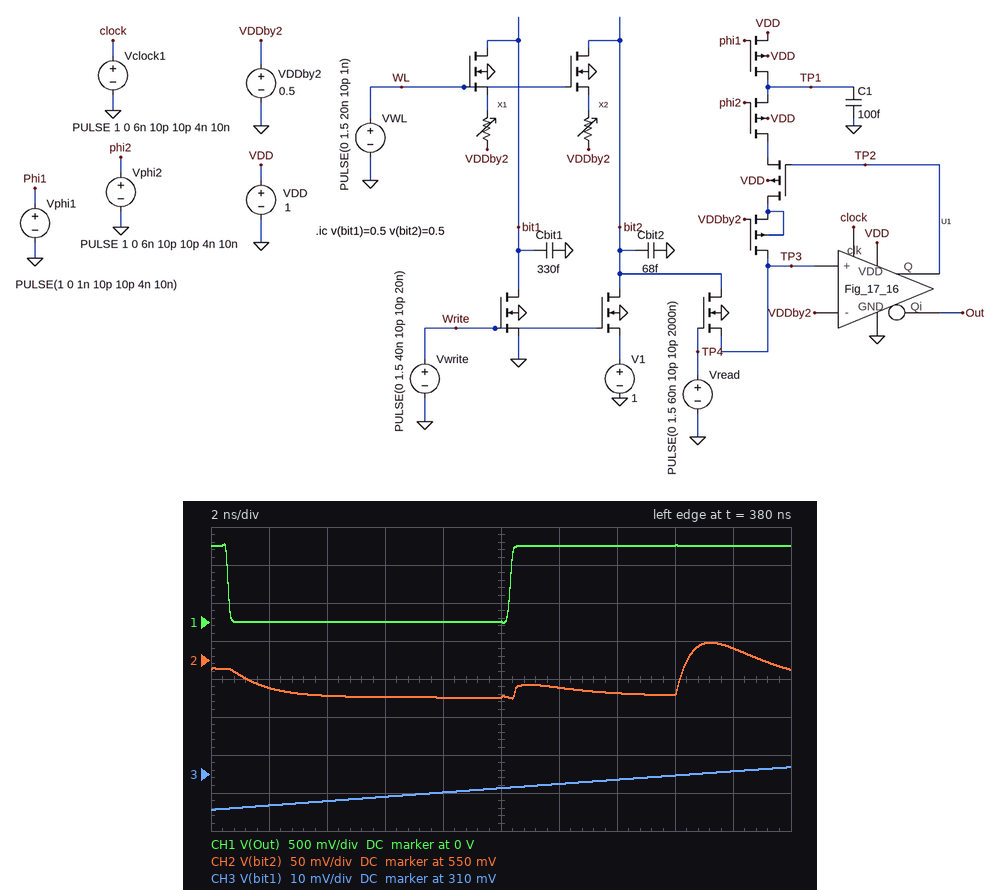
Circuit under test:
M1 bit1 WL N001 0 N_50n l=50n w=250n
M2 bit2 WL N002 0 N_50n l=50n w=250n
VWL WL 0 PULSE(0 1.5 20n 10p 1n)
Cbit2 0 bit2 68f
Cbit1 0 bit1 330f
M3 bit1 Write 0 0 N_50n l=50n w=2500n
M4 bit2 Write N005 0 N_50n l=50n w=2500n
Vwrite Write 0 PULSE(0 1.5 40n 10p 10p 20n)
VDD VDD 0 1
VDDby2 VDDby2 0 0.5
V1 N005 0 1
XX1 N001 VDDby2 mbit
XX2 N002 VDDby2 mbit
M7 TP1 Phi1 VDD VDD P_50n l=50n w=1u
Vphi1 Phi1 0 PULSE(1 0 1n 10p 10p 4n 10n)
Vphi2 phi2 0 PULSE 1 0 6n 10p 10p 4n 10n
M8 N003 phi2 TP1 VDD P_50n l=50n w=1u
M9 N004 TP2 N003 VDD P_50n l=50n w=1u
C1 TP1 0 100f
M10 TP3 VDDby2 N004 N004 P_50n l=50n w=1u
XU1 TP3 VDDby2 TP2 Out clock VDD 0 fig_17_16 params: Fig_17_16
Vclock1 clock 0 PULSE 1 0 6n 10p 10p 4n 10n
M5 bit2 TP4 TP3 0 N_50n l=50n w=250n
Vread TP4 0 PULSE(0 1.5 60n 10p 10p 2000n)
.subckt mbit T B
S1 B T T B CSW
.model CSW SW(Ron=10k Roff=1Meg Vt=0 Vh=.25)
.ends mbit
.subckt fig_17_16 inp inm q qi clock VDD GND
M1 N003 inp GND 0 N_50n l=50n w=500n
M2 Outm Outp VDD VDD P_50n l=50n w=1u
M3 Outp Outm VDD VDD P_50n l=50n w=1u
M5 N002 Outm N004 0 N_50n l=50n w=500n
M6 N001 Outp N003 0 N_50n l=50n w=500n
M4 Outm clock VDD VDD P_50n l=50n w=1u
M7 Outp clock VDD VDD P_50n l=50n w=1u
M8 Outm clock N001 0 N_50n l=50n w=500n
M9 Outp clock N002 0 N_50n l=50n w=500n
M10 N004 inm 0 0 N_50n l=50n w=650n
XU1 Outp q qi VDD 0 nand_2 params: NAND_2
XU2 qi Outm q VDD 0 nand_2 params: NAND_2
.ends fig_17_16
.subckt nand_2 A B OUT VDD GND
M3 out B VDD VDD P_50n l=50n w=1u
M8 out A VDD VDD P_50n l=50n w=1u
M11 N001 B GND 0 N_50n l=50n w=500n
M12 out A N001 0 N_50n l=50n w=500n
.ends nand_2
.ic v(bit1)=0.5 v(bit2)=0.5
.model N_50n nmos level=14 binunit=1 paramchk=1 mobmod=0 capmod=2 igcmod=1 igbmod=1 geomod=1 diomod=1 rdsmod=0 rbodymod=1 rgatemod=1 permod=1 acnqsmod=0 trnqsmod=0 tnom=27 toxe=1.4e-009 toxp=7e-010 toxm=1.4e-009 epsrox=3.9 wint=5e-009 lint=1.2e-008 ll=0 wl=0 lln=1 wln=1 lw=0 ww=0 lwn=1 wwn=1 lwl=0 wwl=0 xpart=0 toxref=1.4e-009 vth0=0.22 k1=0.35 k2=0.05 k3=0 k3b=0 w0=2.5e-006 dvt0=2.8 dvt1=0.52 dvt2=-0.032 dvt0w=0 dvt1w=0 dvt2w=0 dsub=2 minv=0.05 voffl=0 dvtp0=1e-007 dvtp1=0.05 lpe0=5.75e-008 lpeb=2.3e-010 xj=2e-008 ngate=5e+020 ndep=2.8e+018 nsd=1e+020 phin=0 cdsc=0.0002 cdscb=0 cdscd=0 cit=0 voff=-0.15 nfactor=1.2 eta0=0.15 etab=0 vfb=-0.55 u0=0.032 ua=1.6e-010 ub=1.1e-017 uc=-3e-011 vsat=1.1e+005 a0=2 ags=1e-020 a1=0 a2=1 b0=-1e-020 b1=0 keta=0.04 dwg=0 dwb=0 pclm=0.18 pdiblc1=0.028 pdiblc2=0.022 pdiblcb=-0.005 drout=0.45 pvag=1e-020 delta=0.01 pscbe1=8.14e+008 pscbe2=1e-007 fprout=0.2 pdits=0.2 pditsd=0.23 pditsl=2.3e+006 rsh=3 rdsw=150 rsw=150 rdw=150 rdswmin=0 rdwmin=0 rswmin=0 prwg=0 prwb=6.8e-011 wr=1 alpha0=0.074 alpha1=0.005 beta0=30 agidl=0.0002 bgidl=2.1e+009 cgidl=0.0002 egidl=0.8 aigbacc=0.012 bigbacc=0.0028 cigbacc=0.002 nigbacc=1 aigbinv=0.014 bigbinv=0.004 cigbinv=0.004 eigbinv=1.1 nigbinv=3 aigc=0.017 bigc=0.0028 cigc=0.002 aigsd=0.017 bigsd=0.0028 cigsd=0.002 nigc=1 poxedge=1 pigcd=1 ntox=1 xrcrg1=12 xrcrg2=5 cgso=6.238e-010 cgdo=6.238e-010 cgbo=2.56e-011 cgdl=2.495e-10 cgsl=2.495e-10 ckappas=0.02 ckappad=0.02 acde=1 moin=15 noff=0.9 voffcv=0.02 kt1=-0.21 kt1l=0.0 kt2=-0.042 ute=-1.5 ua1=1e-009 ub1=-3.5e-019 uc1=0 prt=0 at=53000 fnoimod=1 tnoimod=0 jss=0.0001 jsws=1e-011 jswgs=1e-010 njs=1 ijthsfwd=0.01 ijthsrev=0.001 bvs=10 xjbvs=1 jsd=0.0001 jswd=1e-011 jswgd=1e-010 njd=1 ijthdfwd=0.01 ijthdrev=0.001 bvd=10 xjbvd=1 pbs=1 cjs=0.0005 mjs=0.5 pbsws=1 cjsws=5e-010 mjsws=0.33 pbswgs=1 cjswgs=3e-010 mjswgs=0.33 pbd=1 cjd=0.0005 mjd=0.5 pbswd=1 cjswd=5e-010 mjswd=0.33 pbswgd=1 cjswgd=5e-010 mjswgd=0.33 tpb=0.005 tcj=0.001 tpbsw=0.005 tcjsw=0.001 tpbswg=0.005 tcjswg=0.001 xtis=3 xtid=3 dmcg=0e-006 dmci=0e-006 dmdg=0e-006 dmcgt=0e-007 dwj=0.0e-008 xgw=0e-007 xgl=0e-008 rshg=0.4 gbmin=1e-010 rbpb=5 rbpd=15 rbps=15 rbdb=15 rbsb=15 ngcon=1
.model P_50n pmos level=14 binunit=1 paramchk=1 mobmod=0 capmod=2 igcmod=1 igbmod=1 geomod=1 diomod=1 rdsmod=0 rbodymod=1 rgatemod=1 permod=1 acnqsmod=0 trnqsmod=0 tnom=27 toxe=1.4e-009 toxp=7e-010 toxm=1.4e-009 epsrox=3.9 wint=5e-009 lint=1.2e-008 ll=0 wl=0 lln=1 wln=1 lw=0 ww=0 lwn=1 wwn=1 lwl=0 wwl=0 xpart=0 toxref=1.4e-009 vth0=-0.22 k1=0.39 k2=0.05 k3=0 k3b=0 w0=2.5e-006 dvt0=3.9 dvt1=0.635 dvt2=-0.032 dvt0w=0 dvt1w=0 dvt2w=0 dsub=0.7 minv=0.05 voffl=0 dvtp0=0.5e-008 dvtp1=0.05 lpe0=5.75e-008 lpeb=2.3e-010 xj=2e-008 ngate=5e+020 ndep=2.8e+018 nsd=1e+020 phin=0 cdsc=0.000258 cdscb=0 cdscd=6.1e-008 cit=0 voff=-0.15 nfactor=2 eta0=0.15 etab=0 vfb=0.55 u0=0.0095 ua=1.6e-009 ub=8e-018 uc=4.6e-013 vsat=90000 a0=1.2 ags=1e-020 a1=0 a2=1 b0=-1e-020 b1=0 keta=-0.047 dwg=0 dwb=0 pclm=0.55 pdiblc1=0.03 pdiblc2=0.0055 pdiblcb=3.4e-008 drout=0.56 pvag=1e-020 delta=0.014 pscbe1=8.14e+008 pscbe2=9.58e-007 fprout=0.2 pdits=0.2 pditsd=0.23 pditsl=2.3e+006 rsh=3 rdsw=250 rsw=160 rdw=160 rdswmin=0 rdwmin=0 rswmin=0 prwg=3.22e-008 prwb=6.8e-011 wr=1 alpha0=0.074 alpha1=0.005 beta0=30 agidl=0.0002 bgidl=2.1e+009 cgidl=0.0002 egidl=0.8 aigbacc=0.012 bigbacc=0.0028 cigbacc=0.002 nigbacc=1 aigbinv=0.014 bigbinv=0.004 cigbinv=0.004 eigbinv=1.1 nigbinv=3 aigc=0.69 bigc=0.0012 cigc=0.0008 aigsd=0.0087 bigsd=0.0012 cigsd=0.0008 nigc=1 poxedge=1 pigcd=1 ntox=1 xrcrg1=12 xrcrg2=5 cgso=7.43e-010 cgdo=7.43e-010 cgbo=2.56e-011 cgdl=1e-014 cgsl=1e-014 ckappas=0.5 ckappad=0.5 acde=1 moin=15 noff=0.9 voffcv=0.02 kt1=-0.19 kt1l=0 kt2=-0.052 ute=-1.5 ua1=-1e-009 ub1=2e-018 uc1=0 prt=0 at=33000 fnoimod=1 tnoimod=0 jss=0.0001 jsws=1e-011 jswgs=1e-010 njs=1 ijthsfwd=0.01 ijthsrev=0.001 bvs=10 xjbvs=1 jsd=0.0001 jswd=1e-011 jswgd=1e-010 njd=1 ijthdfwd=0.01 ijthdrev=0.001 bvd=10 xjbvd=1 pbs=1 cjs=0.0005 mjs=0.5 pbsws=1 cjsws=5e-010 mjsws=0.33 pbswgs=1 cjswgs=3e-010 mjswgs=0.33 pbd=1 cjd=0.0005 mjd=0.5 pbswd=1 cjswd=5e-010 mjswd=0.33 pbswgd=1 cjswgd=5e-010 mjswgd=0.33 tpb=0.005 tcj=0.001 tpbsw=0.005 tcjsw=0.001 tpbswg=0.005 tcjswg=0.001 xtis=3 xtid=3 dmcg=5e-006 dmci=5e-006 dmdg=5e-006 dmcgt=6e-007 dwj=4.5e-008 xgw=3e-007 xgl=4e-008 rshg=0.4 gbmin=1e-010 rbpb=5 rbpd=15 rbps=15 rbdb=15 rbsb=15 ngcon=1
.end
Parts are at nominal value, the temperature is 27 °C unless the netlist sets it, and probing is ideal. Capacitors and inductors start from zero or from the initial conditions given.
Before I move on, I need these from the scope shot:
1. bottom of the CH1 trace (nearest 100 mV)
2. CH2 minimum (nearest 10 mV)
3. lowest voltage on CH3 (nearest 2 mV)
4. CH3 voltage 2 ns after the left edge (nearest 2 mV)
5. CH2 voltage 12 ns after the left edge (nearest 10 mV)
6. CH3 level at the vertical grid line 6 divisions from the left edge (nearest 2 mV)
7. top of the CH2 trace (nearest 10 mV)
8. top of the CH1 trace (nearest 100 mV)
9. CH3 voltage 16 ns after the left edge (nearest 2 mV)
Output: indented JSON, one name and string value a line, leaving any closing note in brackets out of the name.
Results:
{
  "bottom of the CH1 trace": "0 V",
  "CH2 minimum": "500 mV",
  "lowest voltage on CH3": "300 mV",
  "CH3 voltage 2 ns after the left edge": "302 mV",
  "CH2 voltage 12 ns after the left edge": "510 mV",
  "CH3 level at the vertical grid line 6 divisions from the left edge": "308 mV",
  "top of the CH2 trace": "570 mV",
  "top of the CH1 trace": "1.0 V",
  "CH3 voltage 16 ns after the left edge": "310 mV"
}
